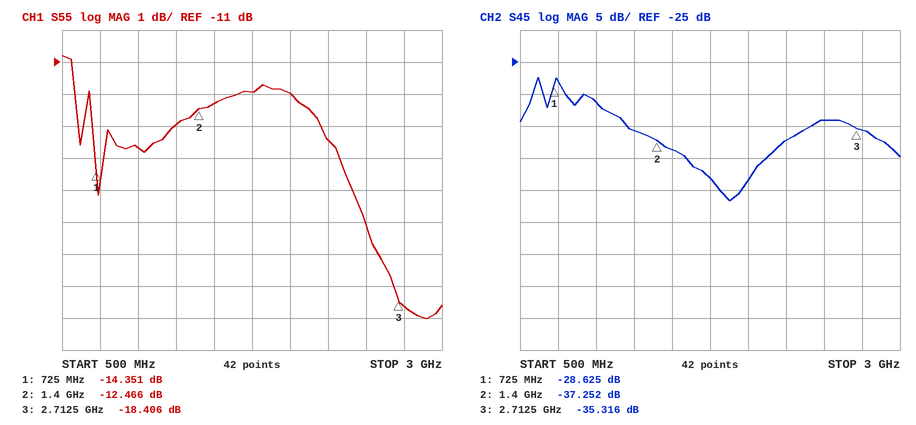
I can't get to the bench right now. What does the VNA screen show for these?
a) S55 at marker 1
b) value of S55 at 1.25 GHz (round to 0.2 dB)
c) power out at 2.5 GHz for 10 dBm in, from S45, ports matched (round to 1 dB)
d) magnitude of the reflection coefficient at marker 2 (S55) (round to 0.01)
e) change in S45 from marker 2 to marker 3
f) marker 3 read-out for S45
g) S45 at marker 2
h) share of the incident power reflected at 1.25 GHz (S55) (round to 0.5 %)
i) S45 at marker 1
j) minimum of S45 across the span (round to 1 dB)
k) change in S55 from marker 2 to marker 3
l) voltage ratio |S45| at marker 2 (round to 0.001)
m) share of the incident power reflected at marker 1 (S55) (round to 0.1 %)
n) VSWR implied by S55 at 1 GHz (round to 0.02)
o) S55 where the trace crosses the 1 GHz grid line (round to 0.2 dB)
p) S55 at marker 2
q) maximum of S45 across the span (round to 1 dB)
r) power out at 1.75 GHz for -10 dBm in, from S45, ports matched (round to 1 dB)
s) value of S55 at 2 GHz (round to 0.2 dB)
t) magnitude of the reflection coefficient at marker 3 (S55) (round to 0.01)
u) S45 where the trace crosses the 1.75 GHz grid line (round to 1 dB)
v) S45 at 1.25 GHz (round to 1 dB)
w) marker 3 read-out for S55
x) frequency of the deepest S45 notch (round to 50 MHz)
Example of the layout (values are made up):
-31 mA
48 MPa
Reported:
-14.351 dB
-13.0 dB
-24 dBm
0.24
1.936 dB
-35.316 dB
-37.252 dB
5.0 %
-28.625 dB
-47 dB
-5.940 dB
0.014
3.7 %
1.52
-13.6 dB
-12.466 dB
-27 dB
-53 dBm
-12.0 dB
0.12
-43 dB
-36 dB
-18.406 dB
1.90 GHz
